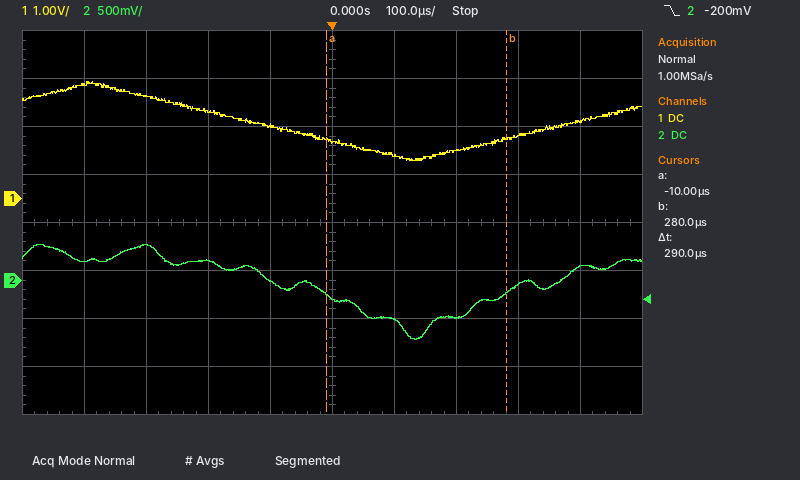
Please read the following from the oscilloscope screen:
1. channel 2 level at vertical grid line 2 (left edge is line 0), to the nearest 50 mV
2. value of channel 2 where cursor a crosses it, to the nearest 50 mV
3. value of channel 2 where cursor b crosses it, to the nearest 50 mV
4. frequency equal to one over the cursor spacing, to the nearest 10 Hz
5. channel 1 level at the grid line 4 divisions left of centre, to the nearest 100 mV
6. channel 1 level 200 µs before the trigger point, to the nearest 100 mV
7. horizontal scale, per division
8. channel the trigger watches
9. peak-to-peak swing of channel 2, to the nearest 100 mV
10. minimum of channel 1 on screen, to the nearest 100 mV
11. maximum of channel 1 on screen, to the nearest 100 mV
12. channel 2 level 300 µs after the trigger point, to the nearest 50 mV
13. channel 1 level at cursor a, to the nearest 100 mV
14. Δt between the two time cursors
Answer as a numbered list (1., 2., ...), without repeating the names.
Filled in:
1. 350 mV
2. -150 mV
3. -150 mV
4. 3.45 kHz
5. 2.4 V
6. 1.8 V
7. 100 µs
8. channel 2
9. 1.00 V
10. 800 mV
11. 2.4 V
12. -50 mV
13. 1.2 V
14. 290 µs
